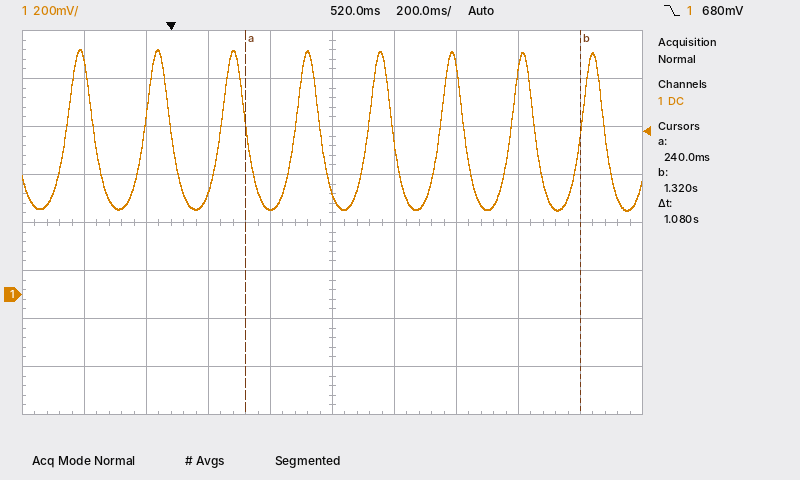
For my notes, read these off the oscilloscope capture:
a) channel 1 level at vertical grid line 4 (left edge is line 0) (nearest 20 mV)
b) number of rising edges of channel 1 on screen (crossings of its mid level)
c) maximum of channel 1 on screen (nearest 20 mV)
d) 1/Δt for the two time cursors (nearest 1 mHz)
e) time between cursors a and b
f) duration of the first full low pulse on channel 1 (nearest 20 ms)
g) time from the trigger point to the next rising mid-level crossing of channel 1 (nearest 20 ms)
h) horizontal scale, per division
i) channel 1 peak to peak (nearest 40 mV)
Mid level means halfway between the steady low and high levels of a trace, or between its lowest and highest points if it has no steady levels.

360 mV
8
1.02 V
926 mHz
1.08 s
160 ms
160 ms
200 ms
680 mV
